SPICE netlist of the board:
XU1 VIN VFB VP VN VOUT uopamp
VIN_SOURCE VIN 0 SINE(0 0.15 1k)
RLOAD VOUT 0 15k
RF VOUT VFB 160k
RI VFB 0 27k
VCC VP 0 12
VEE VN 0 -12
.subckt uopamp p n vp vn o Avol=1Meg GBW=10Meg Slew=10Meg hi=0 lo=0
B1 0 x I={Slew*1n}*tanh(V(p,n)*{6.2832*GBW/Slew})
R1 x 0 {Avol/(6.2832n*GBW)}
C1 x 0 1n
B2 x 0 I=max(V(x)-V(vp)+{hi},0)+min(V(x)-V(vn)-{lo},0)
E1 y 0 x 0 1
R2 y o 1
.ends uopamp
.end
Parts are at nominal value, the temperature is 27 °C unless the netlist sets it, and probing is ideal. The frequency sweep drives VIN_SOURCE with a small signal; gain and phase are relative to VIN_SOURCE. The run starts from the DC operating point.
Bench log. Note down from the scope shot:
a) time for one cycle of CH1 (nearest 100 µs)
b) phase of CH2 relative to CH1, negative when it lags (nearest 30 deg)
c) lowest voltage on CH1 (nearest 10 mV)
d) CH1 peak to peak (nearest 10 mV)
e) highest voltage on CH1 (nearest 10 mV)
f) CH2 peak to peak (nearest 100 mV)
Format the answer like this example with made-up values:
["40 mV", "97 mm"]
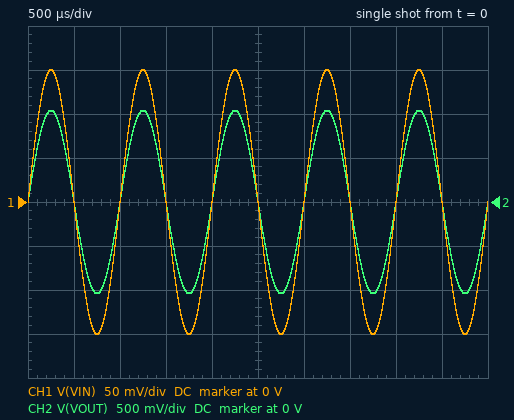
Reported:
["1.0 ms", "0 deg", "-150 mV", "300 mV", "150 mV", "2.1 V"]
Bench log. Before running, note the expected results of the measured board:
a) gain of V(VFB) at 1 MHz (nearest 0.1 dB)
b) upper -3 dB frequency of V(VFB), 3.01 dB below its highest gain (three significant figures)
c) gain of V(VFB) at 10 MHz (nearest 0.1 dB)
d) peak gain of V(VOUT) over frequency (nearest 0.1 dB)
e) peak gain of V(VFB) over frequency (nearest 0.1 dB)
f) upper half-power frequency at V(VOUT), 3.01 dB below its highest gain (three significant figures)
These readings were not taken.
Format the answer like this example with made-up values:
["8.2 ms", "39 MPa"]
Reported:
["-1.7 dB", "1.44 MHz", "-16.9 dB", "16.8 dB", "0 dB", "1.44 MHz"]
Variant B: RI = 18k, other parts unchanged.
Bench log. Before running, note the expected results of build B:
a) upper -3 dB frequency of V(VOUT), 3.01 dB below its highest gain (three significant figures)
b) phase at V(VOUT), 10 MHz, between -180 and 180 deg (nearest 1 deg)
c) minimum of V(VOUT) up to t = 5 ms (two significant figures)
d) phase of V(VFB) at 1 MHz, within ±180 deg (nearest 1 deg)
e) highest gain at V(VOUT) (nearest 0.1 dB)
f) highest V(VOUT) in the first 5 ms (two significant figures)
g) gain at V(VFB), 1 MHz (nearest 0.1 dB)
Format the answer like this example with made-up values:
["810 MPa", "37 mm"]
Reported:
["1.01 MHz", "-84 deg", "-1.5 V", "-45 deg", "19.9 dB", "1.5 V", "-3.0 dB"]
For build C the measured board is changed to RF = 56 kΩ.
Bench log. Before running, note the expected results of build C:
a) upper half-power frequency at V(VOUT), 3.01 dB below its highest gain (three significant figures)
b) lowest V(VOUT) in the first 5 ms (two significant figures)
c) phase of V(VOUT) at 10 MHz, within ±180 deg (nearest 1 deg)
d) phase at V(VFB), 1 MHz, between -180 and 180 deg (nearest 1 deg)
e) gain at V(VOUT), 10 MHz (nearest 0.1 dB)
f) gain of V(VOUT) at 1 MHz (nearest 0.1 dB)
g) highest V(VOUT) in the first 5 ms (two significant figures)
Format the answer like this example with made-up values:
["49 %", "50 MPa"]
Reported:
["3.25 MHz", "-460 mV", "-72 deg", "-17 deg", "-0.4 dB", "9.4 dB", "460 mV"]
